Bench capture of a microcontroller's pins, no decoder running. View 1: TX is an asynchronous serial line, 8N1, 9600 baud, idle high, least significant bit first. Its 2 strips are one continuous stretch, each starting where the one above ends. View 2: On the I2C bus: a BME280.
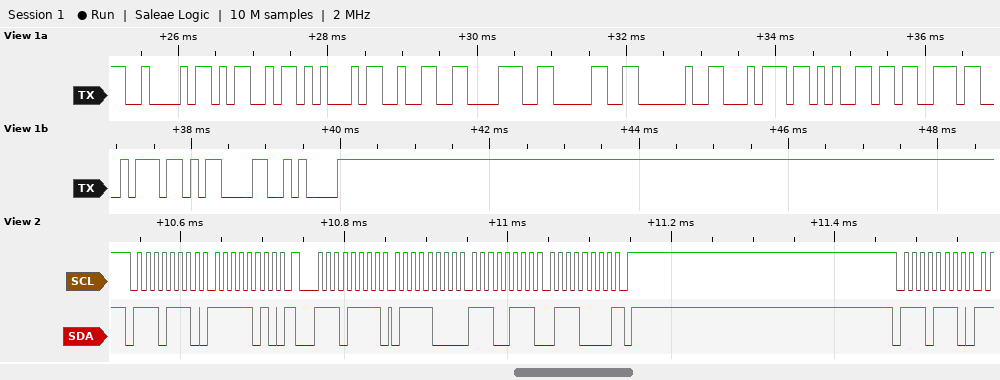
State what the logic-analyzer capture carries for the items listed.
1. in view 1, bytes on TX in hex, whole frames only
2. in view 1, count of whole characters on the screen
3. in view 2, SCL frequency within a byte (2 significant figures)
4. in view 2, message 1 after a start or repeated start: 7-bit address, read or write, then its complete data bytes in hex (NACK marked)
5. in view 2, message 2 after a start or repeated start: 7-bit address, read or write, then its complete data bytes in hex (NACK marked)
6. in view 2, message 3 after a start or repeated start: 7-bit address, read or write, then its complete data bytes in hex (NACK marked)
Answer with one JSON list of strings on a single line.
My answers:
["42 4D 45 32 38 30 20 74 65 73 74 0D 0A", "13", "100 kHz", "0x77 write: FA", "0x77 read: 78 E7 70 NACK", "0x77 write"]
